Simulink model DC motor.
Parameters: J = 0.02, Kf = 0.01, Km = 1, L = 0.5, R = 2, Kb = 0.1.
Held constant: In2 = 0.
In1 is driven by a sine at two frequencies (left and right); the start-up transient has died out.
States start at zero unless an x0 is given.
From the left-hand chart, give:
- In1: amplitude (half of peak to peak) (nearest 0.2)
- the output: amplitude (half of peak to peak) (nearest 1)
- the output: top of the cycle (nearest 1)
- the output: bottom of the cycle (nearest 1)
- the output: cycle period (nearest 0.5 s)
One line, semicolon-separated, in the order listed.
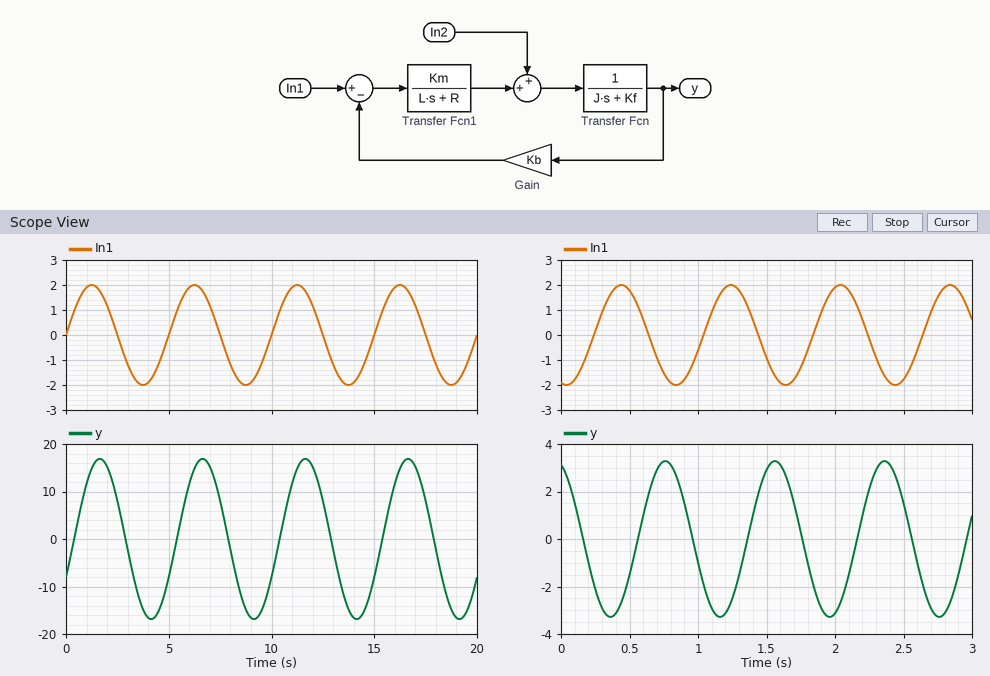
2.0; 17; 17; -17; 5.0 s
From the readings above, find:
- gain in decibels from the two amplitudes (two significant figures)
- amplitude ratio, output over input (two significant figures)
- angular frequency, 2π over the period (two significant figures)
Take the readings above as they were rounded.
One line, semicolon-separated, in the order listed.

19 dB; 8.5; 1.3 rad/s
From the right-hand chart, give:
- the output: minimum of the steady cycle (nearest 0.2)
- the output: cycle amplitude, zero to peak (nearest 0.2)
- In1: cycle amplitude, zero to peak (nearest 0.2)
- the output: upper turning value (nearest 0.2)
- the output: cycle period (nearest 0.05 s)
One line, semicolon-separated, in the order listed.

-3.2; 3.2; 2.0; 3.2; 0.80 s
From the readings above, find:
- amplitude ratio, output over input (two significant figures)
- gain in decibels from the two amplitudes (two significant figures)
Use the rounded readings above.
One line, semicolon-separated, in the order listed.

1.6; 4.1 dB
